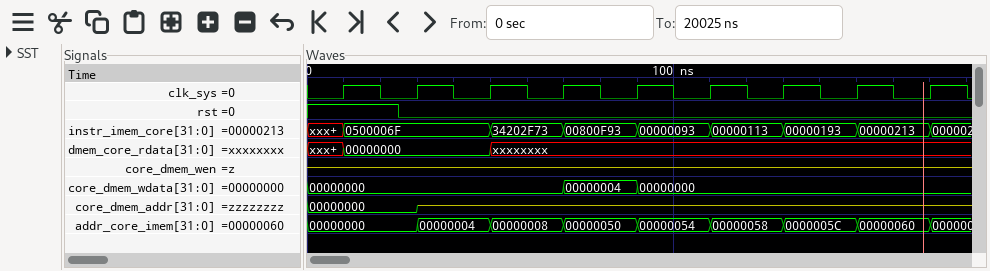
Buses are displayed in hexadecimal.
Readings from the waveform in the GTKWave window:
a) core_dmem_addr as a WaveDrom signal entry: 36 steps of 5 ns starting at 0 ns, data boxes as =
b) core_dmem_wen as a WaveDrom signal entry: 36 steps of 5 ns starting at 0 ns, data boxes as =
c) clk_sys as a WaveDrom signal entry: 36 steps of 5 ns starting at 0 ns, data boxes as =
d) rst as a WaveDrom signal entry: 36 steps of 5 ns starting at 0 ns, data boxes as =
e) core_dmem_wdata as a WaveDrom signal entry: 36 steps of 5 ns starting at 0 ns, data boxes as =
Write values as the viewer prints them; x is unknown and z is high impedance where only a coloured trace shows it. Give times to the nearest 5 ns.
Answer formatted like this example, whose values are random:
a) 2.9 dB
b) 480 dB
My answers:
a) {name: 'core_dmem_addr', wave: '=.....z.............................', data: '00000000'}
b) {name: 'core_dmem_wen', wave: 'z...................................'}
c) {name: 'clk_sys', wave: '0.1.0.1.0.1.0.1.0.1.0.1.0.1.0.1.0.1.'}
d) {name: 'rst', wave: '1....0..............................'}
e) {name: 'core_dmem_wdata', wave: '=.............=...=.................', data: '00000000 00000004 00000000'}
